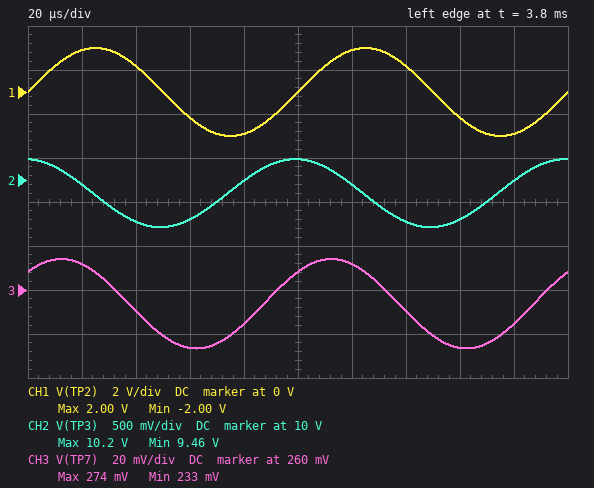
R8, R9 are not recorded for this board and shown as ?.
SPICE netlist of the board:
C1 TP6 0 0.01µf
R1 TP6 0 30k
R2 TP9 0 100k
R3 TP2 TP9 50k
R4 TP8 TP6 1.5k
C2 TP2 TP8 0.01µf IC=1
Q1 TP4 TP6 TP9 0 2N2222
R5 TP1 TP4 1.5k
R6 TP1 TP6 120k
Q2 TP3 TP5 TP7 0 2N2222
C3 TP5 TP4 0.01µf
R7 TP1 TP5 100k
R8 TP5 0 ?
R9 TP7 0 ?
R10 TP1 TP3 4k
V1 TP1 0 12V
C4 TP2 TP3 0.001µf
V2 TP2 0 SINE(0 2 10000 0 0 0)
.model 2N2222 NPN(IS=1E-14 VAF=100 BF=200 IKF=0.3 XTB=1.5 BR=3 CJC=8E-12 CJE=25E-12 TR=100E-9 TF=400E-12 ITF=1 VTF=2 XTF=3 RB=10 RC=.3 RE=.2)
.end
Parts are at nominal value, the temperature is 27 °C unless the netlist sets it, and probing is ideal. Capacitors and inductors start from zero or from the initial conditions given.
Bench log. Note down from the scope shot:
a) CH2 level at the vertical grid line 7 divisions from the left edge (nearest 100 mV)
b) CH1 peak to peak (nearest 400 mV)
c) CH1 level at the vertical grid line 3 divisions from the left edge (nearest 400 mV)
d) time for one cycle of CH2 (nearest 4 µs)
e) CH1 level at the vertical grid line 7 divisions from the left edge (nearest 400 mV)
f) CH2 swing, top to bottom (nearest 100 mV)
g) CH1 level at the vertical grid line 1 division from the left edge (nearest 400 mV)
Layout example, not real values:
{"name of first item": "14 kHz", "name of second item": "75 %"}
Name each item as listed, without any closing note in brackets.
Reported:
{"CH2 level at the vertical grid line 7 divisions from the left edge": "9.5 V", "CH1 peak to peak": "4.0 V", "CH1 level at the vertical grid line 3 divisions from the left edge": "-1.2 V", "time for one cycle of CH2": "100 µs", "CH1 level at the vertical grid line 7 divisions from the left edge": "1.2 V", "CH2 swing, top to bottom": "800 mV", "CH1 level at the vertical grid line 1 division from the left edge": "2.0 V"}
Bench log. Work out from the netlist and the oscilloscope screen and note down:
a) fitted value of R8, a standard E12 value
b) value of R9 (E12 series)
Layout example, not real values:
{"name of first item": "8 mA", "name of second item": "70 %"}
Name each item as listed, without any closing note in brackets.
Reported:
{"fitted value of R8, a standard E12 value": "8.2 kΩ", "value of R9": "470 Ω"}
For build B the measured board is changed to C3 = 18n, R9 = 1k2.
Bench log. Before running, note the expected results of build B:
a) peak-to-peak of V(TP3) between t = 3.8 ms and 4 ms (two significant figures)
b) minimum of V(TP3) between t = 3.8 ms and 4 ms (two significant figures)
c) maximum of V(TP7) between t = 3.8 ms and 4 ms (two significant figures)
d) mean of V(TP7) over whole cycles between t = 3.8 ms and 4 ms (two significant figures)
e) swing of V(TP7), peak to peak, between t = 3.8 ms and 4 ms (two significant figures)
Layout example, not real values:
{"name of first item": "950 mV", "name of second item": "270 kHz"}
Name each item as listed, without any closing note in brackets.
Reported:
{"peak-to-peak of V(TP3) between t = 3.8 ms and 4 ms": "890 mV", "minimum of V(TP3) between t = 3.8 ms and 4 ms": "11 V", "maximum of V(TP7) between t = 3.8 ms and 4 ms": "310 mV", "mean of V(TP7) over whole cycles between t = 3.8 ms and 4 ms": "290 mV", "swing of V(TP7), peak to peak, between t = 3.8 ms and 4 ms": "42 mV"}
